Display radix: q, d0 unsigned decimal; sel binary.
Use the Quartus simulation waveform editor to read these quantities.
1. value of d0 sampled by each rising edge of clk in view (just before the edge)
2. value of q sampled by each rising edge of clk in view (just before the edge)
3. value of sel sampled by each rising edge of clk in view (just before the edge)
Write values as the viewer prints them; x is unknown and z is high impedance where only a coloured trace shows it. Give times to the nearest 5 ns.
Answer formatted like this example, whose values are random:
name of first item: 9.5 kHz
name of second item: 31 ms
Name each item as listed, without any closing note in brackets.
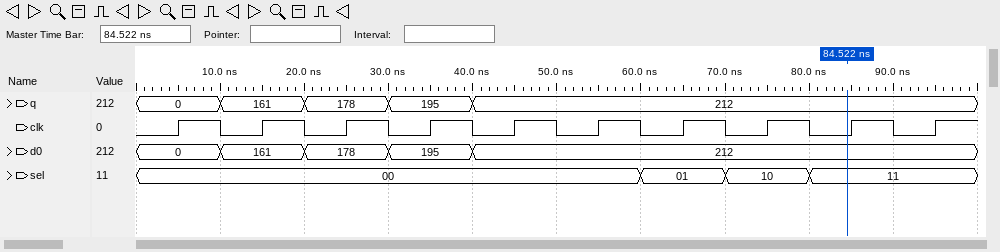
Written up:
value of d0 sampled by each rising edge of clk in view: 0, 161, 178, 195, 212, 212, 212, 212, 212, 212
value of q sampled by each rising edge of clk in view: 0, 161, 178, 195, 212, 212, 212, 212, 212, 212
value of sel sampled by each rising edge of clk in view: 00, 00, 00, 00, 00, 00, 01, 10, 11, 11
